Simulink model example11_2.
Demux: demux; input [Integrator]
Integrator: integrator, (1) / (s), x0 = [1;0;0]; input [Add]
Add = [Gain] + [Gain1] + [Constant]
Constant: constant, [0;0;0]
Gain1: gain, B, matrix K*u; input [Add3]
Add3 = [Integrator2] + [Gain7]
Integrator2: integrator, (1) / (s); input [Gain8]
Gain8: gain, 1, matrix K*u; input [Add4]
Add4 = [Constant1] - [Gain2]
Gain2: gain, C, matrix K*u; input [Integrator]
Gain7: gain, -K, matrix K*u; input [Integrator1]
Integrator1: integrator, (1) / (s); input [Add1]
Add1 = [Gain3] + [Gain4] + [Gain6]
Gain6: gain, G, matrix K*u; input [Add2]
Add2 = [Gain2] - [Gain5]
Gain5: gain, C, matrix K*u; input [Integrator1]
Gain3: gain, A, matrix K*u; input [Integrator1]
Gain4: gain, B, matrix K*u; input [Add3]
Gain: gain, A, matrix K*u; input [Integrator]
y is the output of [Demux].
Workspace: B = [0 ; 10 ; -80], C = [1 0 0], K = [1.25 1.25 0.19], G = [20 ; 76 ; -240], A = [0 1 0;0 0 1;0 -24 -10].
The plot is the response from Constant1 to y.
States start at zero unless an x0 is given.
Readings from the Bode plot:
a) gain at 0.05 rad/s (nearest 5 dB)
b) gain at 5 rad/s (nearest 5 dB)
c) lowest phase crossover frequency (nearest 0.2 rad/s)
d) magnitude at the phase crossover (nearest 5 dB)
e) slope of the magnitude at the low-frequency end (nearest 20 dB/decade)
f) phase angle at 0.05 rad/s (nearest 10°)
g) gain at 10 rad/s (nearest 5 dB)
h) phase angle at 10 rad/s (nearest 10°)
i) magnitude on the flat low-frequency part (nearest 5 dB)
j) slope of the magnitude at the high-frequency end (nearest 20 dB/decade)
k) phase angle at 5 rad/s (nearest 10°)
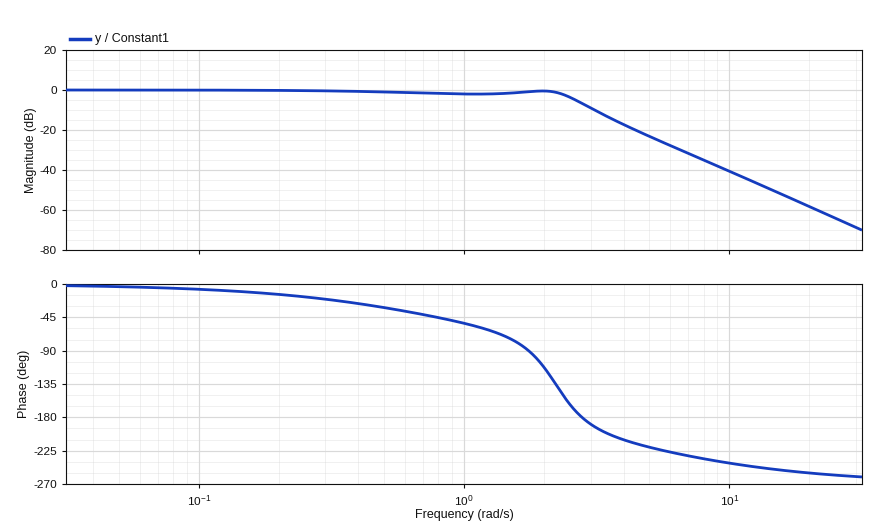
0 dB
-25 dB
2.8 rad/s
-5 dB
0 dB/decade
0°
-40 dB
-240°
0 dB
-60 dB/decade
-220°
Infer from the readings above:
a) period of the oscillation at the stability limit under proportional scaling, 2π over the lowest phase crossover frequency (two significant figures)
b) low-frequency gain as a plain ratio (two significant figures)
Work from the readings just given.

2.2 s
1.0
